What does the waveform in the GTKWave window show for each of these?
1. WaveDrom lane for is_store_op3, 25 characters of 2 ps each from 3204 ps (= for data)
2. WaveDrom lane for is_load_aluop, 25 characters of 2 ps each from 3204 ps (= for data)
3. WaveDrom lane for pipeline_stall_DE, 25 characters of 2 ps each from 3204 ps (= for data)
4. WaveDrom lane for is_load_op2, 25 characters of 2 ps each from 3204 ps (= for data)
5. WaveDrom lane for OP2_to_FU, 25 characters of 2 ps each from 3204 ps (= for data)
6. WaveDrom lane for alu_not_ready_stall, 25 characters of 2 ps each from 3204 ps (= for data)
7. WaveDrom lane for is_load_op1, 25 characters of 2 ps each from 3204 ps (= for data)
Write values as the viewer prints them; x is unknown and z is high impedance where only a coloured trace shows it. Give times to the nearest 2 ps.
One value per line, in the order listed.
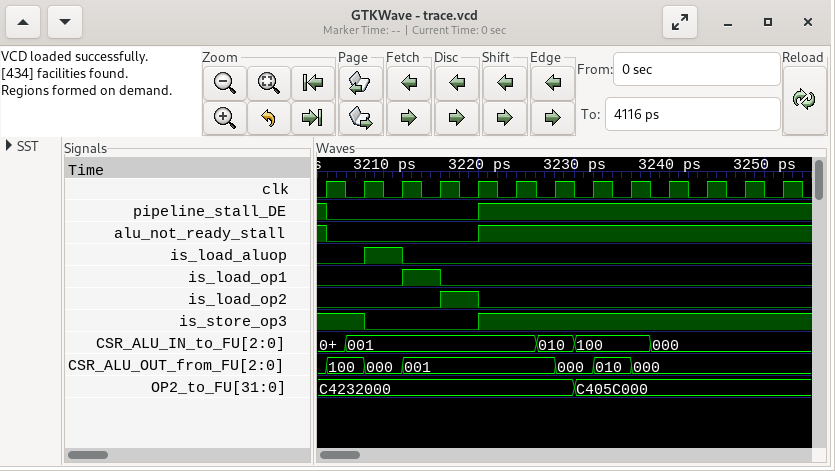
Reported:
{name: 'is_store_op3', wave: '1.0.....1................'}
{name: 'is_load_aluop', wave: '0.1.0....................'}
{name: 'pipeline_stall_DE', wave: '0.......1................'}
{name: 'is_load_op2', wave: '0.....1.0................'}
{name: 'OP2_to_FU', wave: '=............=...........', data: 'C4232000 C405C000'}
{name: 'alu_not_ready_stall', wave: '0.......1................'}
{name: 'is_load_op1', wave: '0...1.0..................'}
